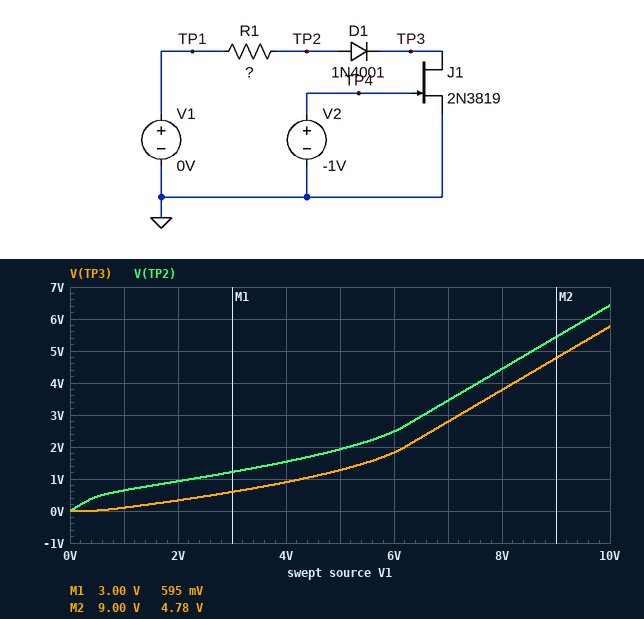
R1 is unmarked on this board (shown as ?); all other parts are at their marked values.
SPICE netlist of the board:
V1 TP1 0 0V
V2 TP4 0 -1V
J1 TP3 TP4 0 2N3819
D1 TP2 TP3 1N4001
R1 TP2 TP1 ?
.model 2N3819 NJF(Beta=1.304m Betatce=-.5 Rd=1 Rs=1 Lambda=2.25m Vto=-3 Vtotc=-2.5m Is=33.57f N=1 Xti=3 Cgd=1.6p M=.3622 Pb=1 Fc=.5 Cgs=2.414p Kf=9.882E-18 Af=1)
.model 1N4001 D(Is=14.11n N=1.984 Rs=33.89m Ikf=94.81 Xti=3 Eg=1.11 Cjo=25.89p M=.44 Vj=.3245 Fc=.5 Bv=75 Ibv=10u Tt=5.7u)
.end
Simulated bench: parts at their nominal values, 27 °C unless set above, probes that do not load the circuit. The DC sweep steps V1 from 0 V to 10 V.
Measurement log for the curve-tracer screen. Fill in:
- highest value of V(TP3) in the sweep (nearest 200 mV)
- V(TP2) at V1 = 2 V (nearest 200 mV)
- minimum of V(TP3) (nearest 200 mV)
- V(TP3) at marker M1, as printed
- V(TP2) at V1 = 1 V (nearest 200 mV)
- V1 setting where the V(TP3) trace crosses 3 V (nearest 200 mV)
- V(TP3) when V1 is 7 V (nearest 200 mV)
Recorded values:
5.8 V
1.0 V
0 V
595 mV
600 mV
7.2 V
2.8 V
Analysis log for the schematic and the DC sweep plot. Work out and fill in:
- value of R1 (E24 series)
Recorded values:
680 Ω
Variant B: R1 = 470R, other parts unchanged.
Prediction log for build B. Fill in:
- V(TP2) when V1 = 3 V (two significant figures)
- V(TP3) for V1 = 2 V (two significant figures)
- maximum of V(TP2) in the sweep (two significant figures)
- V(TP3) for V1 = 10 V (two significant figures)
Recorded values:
1.4 V
440 mV
7.5 V
6.9 V
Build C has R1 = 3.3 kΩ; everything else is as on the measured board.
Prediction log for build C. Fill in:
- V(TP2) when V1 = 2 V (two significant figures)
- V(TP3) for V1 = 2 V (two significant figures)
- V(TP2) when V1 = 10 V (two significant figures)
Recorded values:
610 mV
83 mV
1.2 V
